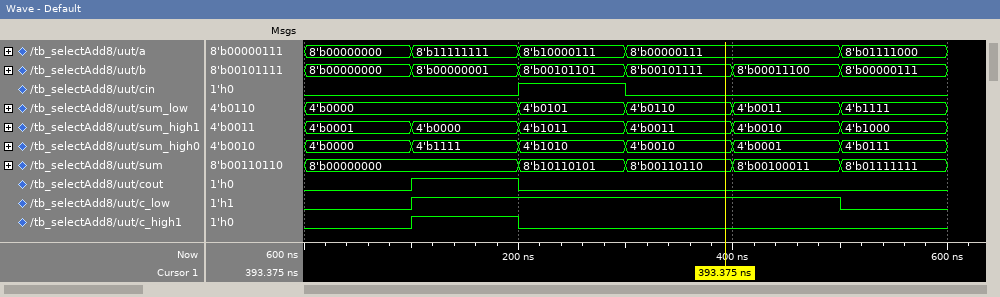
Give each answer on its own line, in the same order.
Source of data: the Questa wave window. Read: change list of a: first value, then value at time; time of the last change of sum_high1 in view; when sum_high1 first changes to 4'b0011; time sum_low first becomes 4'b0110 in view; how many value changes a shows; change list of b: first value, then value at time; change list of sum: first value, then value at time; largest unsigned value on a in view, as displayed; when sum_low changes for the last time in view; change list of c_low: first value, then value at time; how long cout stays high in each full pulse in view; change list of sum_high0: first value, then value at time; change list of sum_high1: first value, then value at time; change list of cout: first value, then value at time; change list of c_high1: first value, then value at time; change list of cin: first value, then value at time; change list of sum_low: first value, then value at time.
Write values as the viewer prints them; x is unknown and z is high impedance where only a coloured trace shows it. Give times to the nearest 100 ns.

8'b00000000, 8'b11111111 at 100 ns, 8'b10000111 at 200 ns, 8'b00000111 at 300 ns, 8'b01111000 at 500 ns
500 ns
300 ns
300 ns
4
8'b00000000, 8'b00000001 at 100 ns, 8'b00101101 at 200 ns, 8'b00101111 at 300 ns, 8'b00011100 at 400 ns, 8'b00000111 at 500 ns
8'b00000000, 8'b10110101 at 200 ns, 8'b00110110 at 300 ns, 8'b00100011 at 400 ns, 8'b01111111 at 500 ns
8'b11111111
500 ns
0, 1 at 100 ns, 0 at 500 ns
100 ns
4'b0000, 4'b1111 at 100 ns, 4'b1010 at 200 ns, 4'b0010 at 300 ns, 4'b0001 at 400 ns, 4'b0111 at 500 ns
4'b0001, 4'b0000 at 100 ns, 4'b1011 at 200 ns, 4'b0011 at 300 ns, 4'b0010 at 400 ns, 4'b1000 at 500 ns
0, 1 at 100 ns, 0 at 200 ns
0, 1 at 100 ns, 0 at 200 ns
0, 1 at 200 ns, 0 at 300 ns
4'b0000, 4'b0101 at 200 ns, 4'b0110 at 300 ns, 4'b0011 at 400 ns, 4'b1111 at 500 ns
